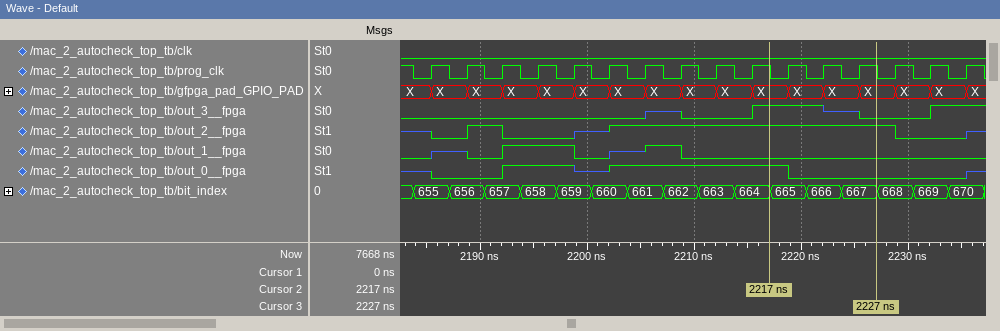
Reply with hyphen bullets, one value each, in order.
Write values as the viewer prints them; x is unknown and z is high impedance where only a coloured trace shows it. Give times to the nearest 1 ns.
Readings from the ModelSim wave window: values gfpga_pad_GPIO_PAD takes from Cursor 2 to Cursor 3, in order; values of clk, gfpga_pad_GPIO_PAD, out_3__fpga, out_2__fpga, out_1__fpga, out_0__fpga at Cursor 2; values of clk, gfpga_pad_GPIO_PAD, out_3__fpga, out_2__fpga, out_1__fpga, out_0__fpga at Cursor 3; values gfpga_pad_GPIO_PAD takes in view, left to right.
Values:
- X, X, X, X
- clk=0, gfpga_pad_GPIO_PAD=X, out_3__fpga=1, out_2__fpga=1, out_1__fpga=0, out_0__fpga=1
- clk=0, gfpga_pad_GPIO_PAD=X, out_3__fpga=0, out_2__fpga=1, out_1__fpga=0, out_0__fpga=0
- X, X, X, X, X, X, X, X, X, X, X, X, X, X, X, X, X
